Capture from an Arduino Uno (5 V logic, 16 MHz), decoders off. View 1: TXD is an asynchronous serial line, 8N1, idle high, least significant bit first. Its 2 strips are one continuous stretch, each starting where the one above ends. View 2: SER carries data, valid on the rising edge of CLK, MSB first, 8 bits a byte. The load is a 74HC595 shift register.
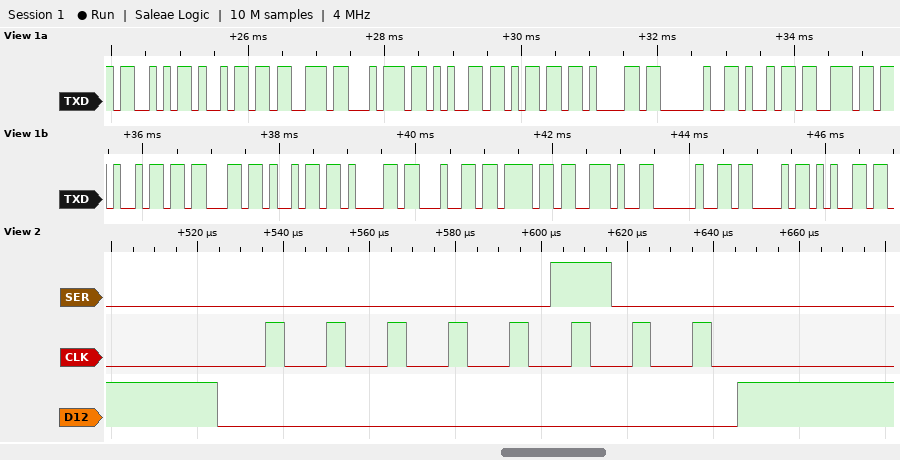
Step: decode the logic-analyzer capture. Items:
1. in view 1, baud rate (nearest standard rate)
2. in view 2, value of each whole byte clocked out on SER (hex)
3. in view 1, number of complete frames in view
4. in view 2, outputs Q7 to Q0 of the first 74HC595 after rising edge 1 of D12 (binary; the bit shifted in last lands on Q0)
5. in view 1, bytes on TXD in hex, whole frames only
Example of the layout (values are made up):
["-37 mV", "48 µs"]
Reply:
["9600 baud", "04", "20", "00000100", "0x53 0x69 0x73 0x74 0x65 0x6D 0x61 0x20 0x69 0x6E 0x69 0x63 0x69 0x61 0x64 0x6F 0x2E 0x20 0x43 0x65"]
